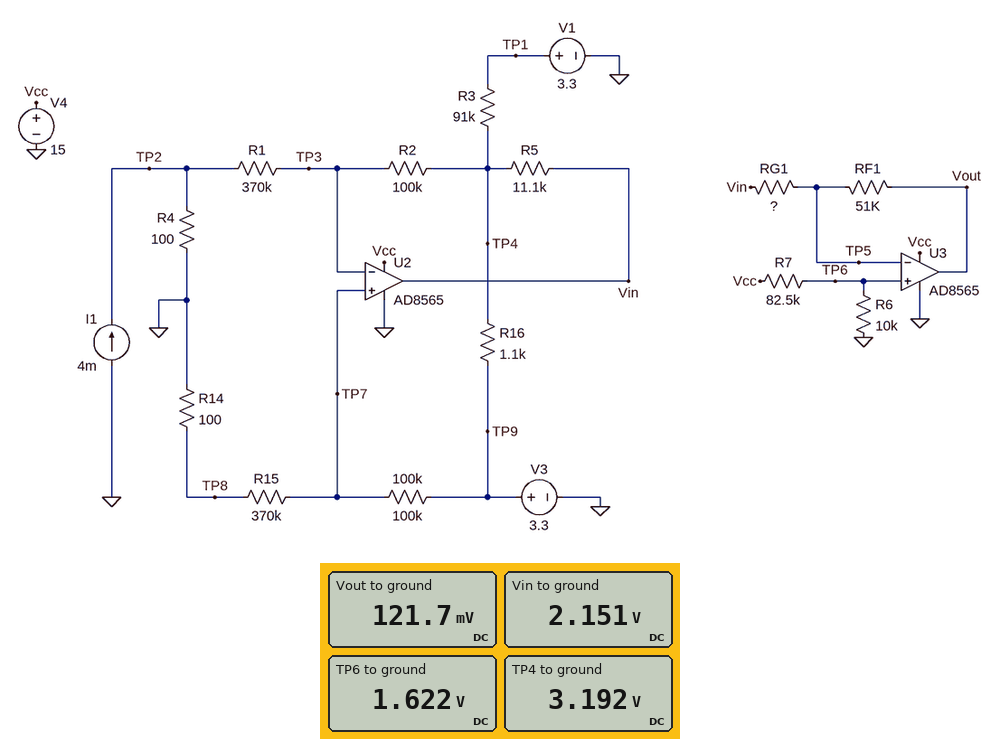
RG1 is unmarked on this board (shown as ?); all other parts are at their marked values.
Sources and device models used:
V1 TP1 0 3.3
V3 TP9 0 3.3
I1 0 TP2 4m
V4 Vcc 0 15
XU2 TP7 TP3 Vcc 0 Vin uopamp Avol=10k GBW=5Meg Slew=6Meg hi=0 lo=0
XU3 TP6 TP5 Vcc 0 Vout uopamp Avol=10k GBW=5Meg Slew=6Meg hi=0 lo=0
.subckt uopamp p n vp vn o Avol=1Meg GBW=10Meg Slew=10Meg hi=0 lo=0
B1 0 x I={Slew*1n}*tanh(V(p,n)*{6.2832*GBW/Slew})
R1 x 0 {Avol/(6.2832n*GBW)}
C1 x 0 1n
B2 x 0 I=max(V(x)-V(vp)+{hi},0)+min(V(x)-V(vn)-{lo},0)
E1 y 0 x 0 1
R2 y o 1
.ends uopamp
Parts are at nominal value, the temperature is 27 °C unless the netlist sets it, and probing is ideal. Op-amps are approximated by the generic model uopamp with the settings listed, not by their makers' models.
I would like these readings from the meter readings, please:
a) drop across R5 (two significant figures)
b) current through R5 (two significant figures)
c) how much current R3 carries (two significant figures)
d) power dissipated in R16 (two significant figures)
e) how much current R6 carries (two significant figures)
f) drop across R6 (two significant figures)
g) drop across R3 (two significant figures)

1.0 V
94 µA
1.2 µA
11 µW
160 µA
1.6 V
110 mV
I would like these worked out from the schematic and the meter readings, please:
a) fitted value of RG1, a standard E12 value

18 kΩ
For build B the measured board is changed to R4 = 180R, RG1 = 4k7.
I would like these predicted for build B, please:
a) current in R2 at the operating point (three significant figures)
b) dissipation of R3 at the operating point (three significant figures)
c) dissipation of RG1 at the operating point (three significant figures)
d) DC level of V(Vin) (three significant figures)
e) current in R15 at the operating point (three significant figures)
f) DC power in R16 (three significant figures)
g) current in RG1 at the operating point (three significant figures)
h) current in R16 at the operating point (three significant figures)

5.07 µA
417 nW
42.9 µW
1.17 V
7.02 µA
34.5 µW
95.5 µA
177 µA
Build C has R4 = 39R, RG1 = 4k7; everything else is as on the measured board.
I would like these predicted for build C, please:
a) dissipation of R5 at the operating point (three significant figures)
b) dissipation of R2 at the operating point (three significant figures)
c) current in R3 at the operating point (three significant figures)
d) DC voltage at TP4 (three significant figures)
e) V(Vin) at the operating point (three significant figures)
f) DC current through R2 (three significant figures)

11.7 µW
4.35 µW
466 nA
3.26 V
2.90 V
6.60 µA
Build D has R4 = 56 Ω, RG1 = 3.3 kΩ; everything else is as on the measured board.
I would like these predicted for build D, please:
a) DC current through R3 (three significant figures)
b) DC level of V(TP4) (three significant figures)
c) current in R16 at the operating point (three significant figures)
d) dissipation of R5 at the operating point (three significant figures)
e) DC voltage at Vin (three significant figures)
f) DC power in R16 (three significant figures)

668 nA
3.24 V
55.3 µA
27.2 µW
2.69 V
3.36 µW
